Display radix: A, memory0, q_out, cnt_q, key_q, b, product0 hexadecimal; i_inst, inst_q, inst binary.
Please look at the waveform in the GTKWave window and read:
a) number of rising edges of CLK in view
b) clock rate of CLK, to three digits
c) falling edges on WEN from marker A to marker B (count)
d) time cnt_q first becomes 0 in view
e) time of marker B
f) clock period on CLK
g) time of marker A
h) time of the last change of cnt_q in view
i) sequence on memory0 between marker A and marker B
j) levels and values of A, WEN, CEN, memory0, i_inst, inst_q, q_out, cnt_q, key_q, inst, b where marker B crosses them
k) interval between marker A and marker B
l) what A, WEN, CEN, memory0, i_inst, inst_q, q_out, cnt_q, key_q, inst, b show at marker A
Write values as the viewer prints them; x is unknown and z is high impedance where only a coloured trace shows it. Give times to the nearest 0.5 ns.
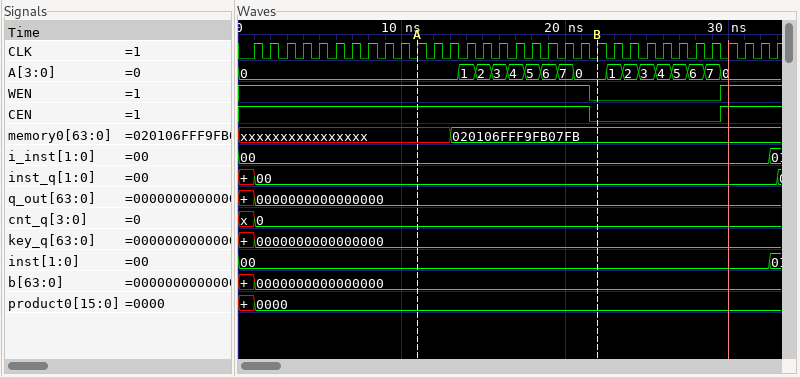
33
1.00 GHz
1
1 ns
22 ns
1 ns
11 ns
1 ns
xxxxxxxxxxxxxxxx, 020106FFF9FB07FB
A=0, WEN=0, CEN=0, memory0=020106FFF9FB07FB, i_inst=00, inst_q=00, q_out=0000000000000000, cnt_q=0, key_q=0000000000000000, inst=00, b=0000000000000000
11 ns
A=0, WEN=1, CEN=1, memory0=xxxxxxxxxxxxxxxx, i_inst=00, inst_q=00, q_out=0000000000000000, cnt_q=0, key_q=0000000000000000, inst=00, b=0000000000000000
